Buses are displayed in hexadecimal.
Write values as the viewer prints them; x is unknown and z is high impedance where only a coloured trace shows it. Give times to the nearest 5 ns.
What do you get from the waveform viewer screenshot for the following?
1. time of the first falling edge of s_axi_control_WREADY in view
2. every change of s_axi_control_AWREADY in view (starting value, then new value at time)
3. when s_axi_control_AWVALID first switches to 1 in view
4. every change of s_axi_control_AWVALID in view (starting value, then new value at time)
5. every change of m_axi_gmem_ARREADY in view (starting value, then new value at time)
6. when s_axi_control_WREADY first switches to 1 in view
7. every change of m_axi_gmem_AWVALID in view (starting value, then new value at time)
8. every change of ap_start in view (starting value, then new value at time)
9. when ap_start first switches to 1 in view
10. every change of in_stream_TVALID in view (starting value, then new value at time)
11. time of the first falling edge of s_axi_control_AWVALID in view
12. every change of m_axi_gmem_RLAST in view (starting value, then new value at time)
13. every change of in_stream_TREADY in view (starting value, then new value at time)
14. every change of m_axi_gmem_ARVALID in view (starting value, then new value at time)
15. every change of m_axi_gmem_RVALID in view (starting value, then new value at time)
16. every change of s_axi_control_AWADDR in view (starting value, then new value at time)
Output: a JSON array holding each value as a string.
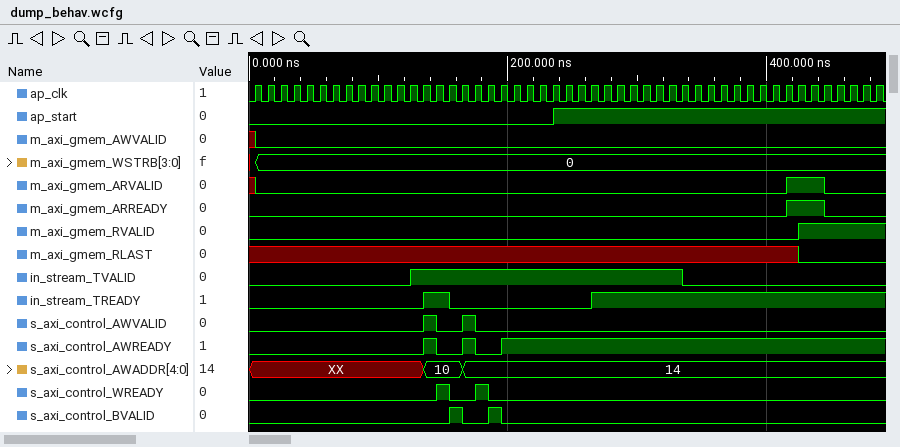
["155 ns", "0, 1 at 135 ns, 0 at 145 ns, 1 at 165 ns, 0 at 175 ns, 1 at 195 ns", "135 ns", "0, 1 at 135 ns, 0 at 145 ns, 1 at 165 ns, 0 at 175 ns", "0, 1 at 415 ns, 0 at 445 ns", "145 ns", "x, 0 at 5 ns", "0, 1 at 235 ns", "235 ns", "0, 1 at 125 ns, 0 at 335 ns", "145 ns", "x, 0 at 425 ns", "0, 1 at 135 ns, 0 at 155 ns, 1 at 265 ns", "x, 0 at 5 ns, 1 at 415 ns, 0 at 445 ns", "0, 1 at 425 ns", "XX, 10 at 135 ns, 14 at 165 ns"]
